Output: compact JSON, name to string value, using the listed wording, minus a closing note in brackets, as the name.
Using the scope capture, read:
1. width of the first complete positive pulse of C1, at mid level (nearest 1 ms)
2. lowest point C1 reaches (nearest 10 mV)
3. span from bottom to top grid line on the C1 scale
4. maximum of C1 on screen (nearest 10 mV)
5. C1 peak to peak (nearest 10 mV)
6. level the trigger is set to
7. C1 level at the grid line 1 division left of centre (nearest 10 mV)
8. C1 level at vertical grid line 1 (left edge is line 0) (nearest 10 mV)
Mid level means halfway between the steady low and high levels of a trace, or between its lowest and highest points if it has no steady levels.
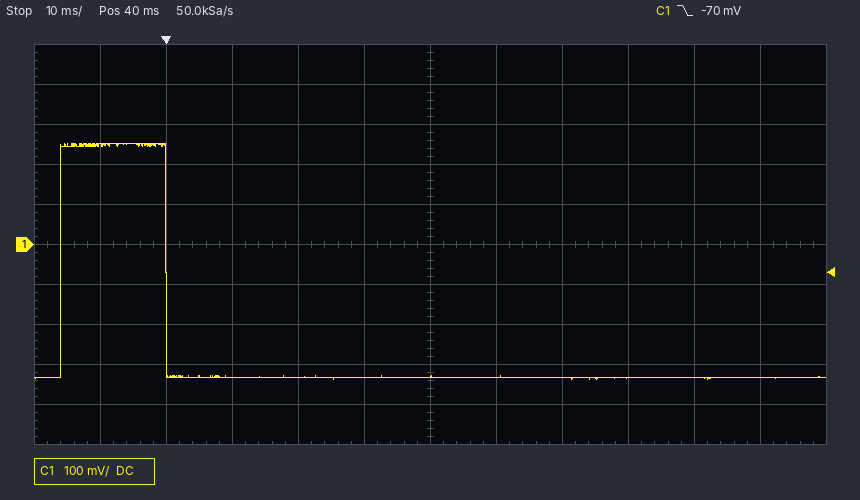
{"width of the first complete positive pulse of C1, at mid level": "16 ms", "lowest point C1 reaches": "-340 mV", "span from bottom to top grid line on the C1 scale": "1 V", "maximum of C1 on screen": "250 mV", "C1 peak to peak": "590 mV", "level the trigger is set to": "-70 mV", "C1 level at the grid line 1 division left of centre": "-330 mV", "C1 level at vertical grid line 1 (left edge is line 0)": "250 mV"}
